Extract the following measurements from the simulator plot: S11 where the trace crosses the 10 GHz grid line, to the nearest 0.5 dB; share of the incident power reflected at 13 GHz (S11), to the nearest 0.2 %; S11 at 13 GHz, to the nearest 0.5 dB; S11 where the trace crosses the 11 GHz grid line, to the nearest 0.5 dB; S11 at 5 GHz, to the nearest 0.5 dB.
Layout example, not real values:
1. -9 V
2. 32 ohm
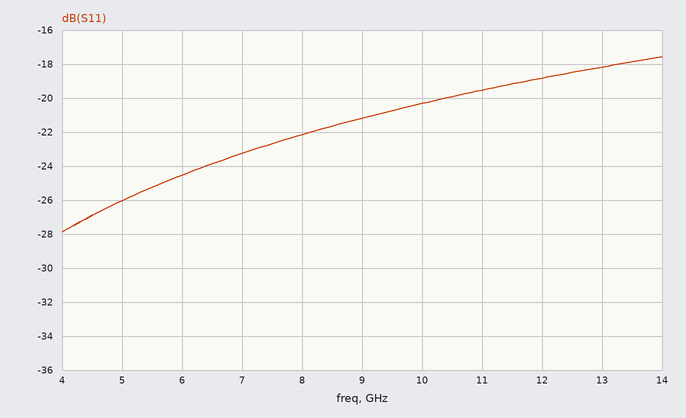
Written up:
1. -20.5 dB
2. 1.6 %
3. -18.0 dB
4. -19.5 dB
5. -26.0 dB
